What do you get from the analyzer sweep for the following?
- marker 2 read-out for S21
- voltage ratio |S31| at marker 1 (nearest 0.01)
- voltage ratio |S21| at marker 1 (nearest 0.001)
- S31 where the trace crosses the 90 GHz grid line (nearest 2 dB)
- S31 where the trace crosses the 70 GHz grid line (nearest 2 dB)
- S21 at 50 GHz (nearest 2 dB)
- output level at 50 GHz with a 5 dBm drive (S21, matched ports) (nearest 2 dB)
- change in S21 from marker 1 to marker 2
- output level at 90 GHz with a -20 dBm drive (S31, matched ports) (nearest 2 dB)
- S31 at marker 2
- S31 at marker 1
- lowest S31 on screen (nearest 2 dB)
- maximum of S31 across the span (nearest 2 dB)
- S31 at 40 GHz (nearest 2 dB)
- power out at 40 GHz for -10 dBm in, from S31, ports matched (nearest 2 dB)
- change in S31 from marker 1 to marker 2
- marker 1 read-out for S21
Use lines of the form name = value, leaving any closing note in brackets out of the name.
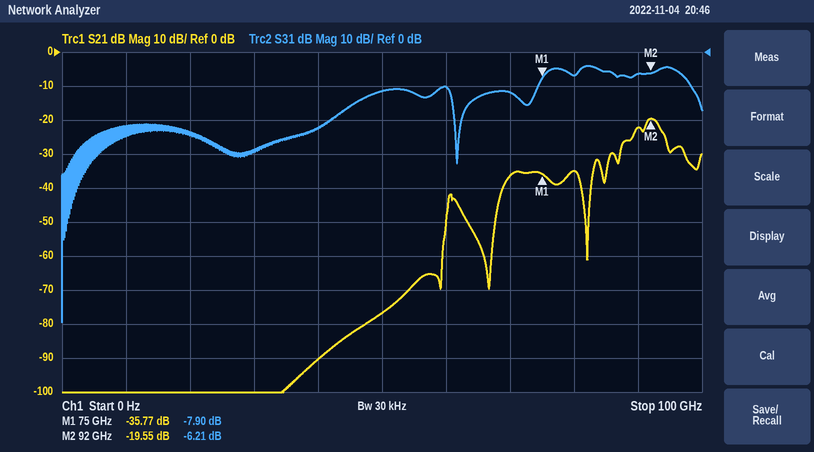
marker 2 read-out for S21 = -19.55 dB
voltage ratio |S31| at marker 1 = 0.40
voltage ratio |S21| at marker 1 = 0.016
S31 where the trace crosses the 90 GHz grid line = -6 dB
S31 where the trace crosses the 70 GHz grid line = -12 dB
S21 at 50 GHz = -76 dB
output level at 50 GHz with a 5 dBm drive (S21, matched ports) = -72 dBm
change in S21 from marker 1 to marker 2 = 16.22 dB
output level at 90 GHz with a -20 dBm drive (S31, matched ports) = -26 dBm
S31 at marker 2 = -6.21 dB
S31 at marker 1 = -7.90 dB
lowest S31 on screen = -80 dB
maximum of S31 across the span = -4 dB
S31 at 40 GHz = -22 dB
power out at 40 GHz for -10 dBm in, from S31, ports matched = -32 dBm
change in S31 from marker 1 to marker 2 = 1.69 dB
marker 1 read-out for S21 = -35.77 dB
